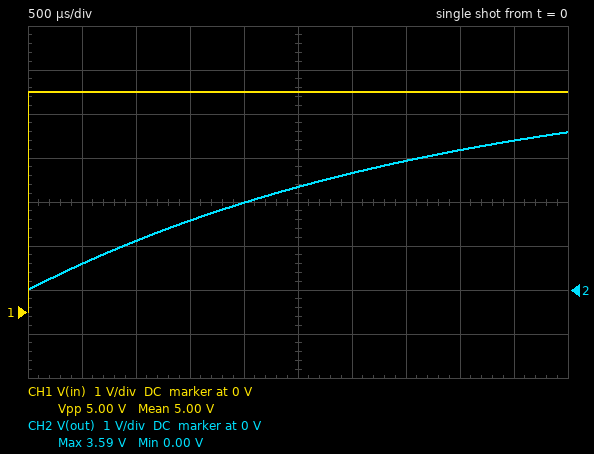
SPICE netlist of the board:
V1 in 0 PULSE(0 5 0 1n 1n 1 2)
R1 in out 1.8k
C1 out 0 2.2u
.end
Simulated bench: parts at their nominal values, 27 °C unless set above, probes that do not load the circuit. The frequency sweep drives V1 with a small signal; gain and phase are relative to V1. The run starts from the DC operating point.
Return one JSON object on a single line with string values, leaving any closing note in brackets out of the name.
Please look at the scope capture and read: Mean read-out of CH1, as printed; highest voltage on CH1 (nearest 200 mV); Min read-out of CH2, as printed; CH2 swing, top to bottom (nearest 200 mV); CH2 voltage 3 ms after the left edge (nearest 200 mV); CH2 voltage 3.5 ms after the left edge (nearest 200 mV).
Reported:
{"Mean read-out of CH1, as printed": "5.00 V", "highest voltage on CH1": "5.0 V", "Min read-out of CH2, as printed": "0.00 V", "CH2 swing, top to bottom": "3.6 V", "CH2 voltage 3 ms after the left edge": "2.6 V", "CH2 voltage 3.5 ms after the left edge": "3.0 V"}
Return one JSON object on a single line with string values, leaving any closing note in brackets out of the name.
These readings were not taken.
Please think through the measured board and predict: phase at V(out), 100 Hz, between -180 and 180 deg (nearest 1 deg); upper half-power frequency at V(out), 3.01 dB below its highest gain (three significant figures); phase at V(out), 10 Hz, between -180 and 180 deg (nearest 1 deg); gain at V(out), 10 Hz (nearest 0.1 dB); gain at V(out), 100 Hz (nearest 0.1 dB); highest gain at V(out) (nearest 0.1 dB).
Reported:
{"phase at V(out), 100 Hz, between -180 and 180 deg": "-68 deg", "upper half-power frequency at V(out), 3.01 dB below its highest gain": "40.2 Hz", "phase at V(out), 10 Hz, between -180 and 180 deg": "-14 deg", "gain at V(out), 10 Hz": "-0.3 dB", "gain at V(out), 100 Hz": "-8.6 dB", "highest gain at V(out)": "0 dB"}
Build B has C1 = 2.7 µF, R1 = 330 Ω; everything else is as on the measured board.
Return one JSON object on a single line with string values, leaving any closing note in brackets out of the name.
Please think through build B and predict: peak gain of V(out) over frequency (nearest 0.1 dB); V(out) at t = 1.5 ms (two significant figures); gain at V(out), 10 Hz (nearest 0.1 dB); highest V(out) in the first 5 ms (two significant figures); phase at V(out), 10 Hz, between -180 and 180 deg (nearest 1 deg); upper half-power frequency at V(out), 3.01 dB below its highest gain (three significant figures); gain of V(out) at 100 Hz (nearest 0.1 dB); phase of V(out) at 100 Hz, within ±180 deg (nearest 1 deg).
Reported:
{"peak gain of V(out) over frequency": "0 dB", "V(out) at t = 1.5 ms": "4.1 V", "gain at V(out), 10 Hz": "0 dB", "highest V(out) in the first 5 ms": "5.0 V", "phase at V(out), 10 Hz, between -180 and 180 deg": "-3 deg", "upper half-power frequency at V(out), 3.01 dB below its highest gain": "179 Hz", "gain of V(out) at 100 Hz": "-1.2 dB", "phase of V(out) at 100 Hz, within ±180 deg": "-29 deg"}
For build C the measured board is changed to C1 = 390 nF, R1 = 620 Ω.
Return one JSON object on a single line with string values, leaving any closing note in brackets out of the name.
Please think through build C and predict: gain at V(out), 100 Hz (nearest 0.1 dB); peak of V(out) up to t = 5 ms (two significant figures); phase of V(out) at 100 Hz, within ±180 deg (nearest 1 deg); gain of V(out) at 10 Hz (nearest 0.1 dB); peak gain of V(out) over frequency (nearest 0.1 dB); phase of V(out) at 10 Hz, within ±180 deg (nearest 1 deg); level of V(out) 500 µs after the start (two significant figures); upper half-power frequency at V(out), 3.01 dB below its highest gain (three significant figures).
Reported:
{"gain at V(out), 100 Hz": "-0.1 dB", "peak of V(out) up to t = 5 ms": "5.0 V", "phase of V(out) at 100 Hz, within ±180 deg": "-9 deg", "gain of V(out) at 10 Hz": "0 dB", "peak gain of V(out) over frequency": "0 dB", "phase of V(out) at 10 Hz, within ±180 deg": "-1 deg", "level of V(out) 500 µs after the start": "4.4 V", "upper half-power frequency at V(out), 3.01 dB below its highest gain": "658 Hz"}
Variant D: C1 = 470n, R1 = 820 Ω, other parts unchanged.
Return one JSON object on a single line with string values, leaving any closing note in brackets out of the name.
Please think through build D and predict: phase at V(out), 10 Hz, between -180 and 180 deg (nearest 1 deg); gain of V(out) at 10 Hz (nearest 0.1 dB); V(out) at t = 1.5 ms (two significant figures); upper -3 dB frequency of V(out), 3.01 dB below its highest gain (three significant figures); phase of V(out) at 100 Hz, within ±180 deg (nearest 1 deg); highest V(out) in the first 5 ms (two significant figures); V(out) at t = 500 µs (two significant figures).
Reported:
{"phase at V(out), 10 Hz, between -180 and 180 deg": "-1 deg", "gain of V(out) at 10 Hz": "0 dB", "V(out) at t = 1.5 ms": "4.9 V", "upper -3 dB frequency of V(out), 3.01 dB below its highest gain": "413 Hz", "phase of V(out) at 100 Hz, within ±180 deg": "-14 deg", "highest V(out) in the first 5 ms": "5.0 V", "V(out) at t = 500 µs": "3.6 V"}
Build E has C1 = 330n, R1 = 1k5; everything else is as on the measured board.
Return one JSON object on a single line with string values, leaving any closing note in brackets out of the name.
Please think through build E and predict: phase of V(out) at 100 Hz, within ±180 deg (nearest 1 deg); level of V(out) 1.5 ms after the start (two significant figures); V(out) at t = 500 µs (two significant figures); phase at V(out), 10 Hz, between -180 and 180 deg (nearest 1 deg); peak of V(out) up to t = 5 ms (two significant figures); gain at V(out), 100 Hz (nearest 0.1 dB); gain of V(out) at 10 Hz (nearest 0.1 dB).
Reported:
{"phase of V(out) at 100 Hz, within ±180 deg": "-17 deg", "level of V(out) 1.5 ms after the start": "4.8 V", "V(out) at t = 500 µs": "3.2 V", "phase at V(out), 10 Hz, between -180 and 180 deg": "-2 deg", "peak of V(out) up to t = 5 ms": "5.0 V", "gain at V(out), 100 Hz": "-0.4 dB", "gain of V(out) at 10 Hz": "0 dB"}
